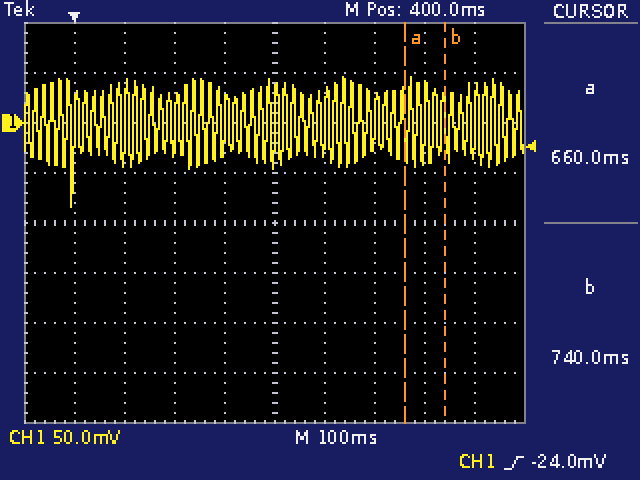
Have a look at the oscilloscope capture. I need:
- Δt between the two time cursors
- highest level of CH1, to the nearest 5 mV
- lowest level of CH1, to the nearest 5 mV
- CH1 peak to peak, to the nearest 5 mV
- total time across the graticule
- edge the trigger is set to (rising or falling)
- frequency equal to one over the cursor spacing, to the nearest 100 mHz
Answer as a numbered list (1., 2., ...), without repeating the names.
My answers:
1. 80 ms
2. 45 mV
3. -85 mV
4. 130 mV
5. 1 s
6. rising
7. 12.5 Hz
